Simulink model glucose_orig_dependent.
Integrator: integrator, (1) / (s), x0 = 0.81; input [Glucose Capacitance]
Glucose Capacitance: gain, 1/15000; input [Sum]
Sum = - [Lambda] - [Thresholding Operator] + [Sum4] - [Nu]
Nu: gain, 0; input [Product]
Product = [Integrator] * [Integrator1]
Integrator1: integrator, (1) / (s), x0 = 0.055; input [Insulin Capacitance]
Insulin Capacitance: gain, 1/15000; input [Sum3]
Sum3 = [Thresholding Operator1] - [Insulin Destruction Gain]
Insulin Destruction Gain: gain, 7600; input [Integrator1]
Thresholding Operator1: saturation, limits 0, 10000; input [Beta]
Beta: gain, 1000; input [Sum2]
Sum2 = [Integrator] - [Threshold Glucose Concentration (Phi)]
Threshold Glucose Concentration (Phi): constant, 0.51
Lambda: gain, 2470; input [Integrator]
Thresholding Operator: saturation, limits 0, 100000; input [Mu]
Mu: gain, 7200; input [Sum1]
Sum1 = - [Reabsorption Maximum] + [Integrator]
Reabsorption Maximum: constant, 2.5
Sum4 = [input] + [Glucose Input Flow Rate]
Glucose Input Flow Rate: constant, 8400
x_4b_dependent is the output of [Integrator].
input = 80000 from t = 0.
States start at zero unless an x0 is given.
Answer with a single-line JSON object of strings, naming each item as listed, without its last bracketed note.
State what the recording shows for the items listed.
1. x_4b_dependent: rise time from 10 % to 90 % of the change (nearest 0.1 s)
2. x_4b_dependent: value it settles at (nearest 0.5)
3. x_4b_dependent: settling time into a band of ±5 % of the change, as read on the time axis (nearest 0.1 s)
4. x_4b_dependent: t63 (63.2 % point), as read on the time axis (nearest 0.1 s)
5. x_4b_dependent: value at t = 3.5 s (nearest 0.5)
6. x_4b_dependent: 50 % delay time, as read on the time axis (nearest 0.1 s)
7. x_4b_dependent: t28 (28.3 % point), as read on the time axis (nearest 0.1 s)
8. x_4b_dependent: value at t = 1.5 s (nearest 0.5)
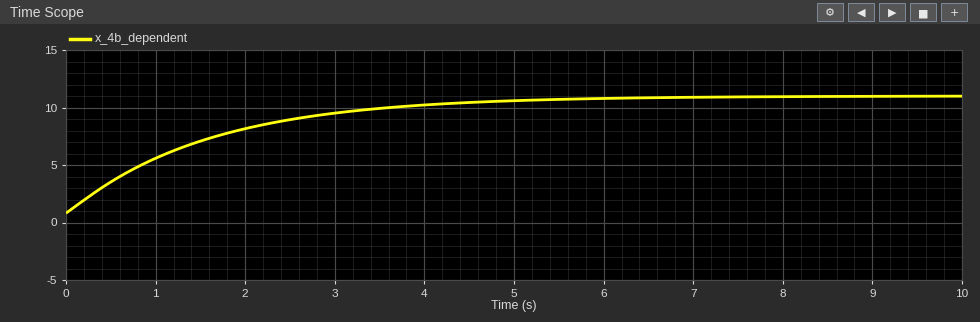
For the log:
{"x_4b_dependent: rise time from 10 % to 90 % of the change": "3.4 s", "x_4b_dependent: value it settles at": "11.0", "x_4b_dependent: settling time into a band of ±5 % of the change, as read on the time axis": "4.7 s", "x_4b_dependent: t63 (63.2 % point), as read on the time axis": "1.6 s", "x_4b_dependent: value at t = 3.5 s": "10.0", "x_4b_dependent: 50 % delay time, as read on the time axis": "1.1 s", "x_4b_dependent: t28 (28.3 % point), as read on the time axis": "0.5 s", "x_4b_dependent: value at t = 1.5 s": "7.0"}
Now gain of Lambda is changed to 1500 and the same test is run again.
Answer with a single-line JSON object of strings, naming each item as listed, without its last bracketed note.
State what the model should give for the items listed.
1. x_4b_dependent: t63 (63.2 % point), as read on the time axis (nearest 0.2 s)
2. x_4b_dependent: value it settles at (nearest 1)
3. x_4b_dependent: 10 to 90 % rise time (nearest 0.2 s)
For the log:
{"x_4b_dependent: t63 (63.2 % point), as read on the time axis": "1.8 s", "x_4b_dependent: value it settles at": "12", "x_4b_dependent: 10 to 90 % rise time": "3.8 s"}
